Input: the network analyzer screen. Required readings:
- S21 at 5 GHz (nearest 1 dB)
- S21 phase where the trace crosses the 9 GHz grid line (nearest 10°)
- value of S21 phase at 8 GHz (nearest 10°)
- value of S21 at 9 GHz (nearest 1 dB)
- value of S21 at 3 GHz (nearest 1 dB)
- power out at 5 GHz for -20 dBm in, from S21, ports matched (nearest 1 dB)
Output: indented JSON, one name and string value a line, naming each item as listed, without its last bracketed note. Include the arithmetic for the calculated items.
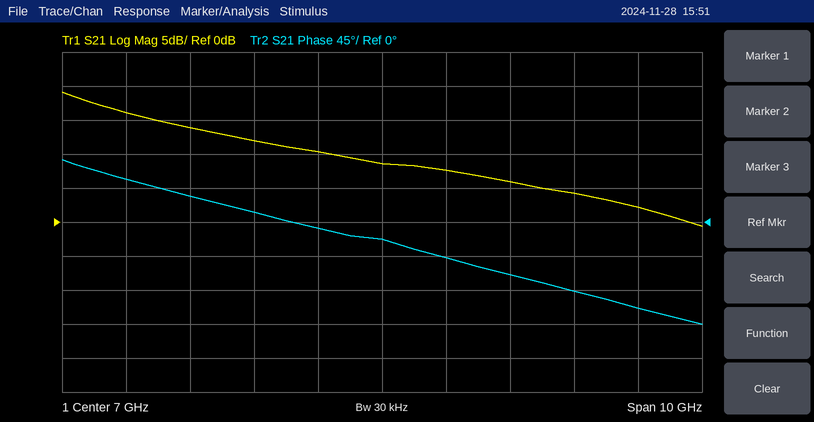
{
  "S21 at 5 GHz": "12 dB",
  "S21 phase where the trace crosses the 9 GHz grid line": "-70°",
  "value of S21 phase at 8 GHz": "-50°",
  "value of S21 at 9 GHz": "6 dB",
  "value of S21 at 3 GHz": "16 dB",
  "power out at 5 GHz for -20 dBm in, from S21, ports matched": "-20 dBm + (12 dB) = -8 dBm"
}
